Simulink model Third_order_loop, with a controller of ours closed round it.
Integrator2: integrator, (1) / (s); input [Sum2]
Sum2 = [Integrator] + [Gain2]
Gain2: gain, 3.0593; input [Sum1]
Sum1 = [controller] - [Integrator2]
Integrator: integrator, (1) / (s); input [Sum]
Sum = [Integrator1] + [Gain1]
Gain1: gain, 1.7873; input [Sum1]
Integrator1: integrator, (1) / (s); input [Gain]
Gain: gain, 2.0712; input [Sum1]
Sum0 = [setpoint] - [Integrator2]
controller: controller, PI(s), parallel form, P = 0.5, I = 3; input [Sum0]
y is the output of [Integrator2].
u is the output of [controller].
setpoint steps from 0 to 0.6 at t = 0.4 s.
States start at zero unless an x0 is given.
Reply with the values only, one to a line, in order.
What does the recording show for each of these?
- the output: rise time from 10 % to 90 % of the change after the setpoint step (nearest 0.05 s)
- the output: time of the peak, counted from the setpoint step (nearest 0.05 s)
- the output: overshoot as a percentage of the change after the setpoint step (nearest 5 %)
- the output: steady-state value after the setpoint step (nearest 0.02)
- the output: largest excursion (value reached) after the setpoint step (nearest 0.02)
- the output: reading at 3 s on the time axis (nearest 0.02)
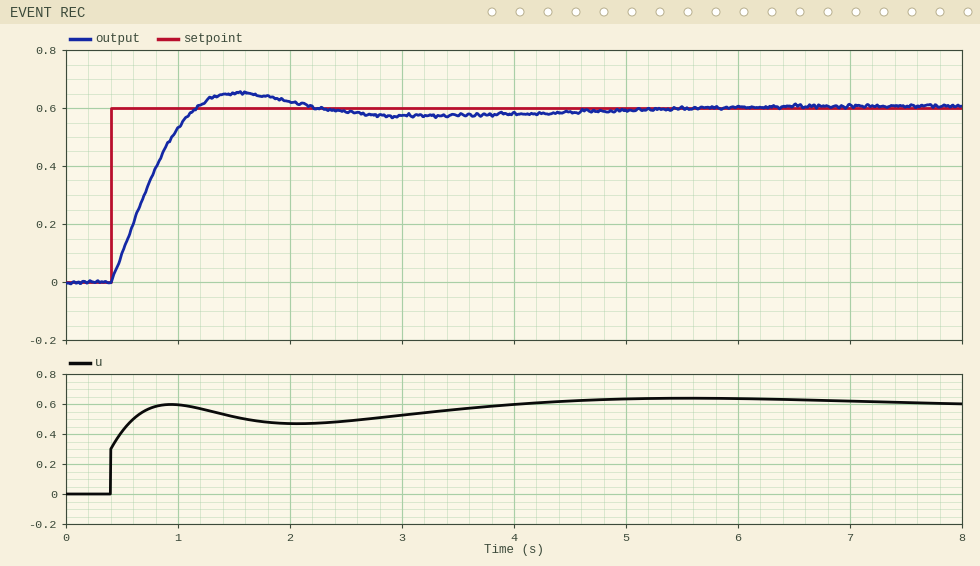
0.55 s
1.15 s
10 %
0.60
0.66
0.58
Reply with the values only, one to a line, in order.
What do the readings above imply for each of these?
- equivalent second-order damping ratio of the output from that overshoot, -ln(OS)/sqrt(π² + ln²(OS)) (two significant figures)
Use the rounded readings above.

0.59
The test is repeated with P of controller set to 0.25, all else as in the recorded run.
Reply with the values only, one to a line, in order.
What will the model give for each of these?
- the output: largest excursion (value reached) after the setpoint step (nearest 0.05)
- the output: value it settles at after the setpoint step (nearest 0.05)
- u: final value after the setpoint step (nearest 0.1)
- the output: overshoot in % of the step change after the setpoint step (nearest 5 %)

0.70
0.60
0.6
15 %
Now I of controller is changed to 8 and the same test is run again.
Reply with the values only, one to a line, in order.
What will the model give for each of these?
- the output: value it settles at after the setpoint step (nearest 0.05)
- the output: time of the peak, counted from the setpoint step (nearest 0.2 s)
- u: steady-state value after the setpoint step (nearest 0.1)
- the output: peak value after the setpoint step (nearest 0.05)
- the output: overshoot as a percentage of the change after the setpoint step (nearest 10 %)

0.60
0.6 s
0.6
0.75
30 %
